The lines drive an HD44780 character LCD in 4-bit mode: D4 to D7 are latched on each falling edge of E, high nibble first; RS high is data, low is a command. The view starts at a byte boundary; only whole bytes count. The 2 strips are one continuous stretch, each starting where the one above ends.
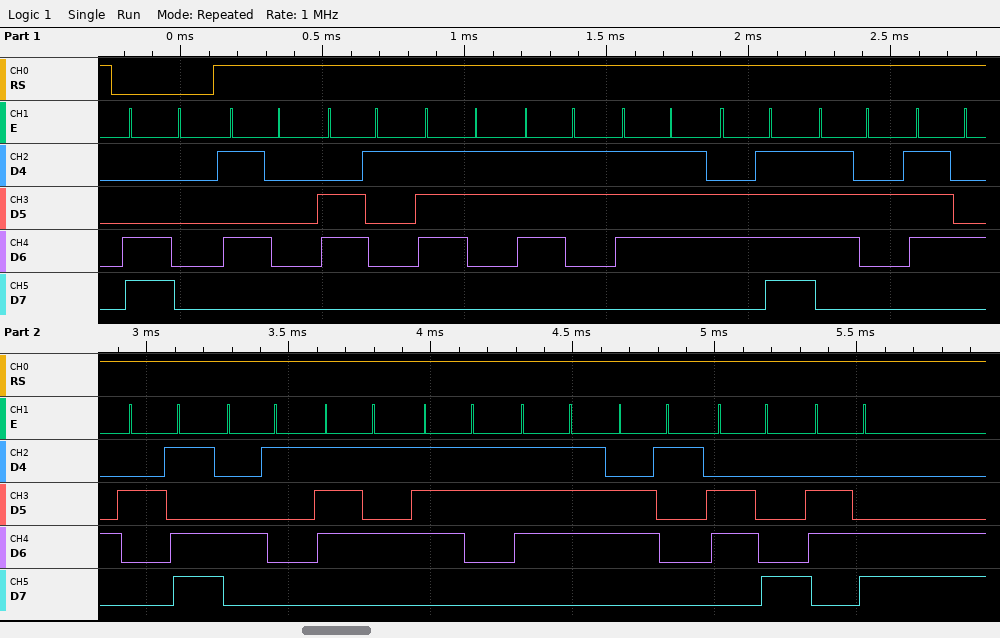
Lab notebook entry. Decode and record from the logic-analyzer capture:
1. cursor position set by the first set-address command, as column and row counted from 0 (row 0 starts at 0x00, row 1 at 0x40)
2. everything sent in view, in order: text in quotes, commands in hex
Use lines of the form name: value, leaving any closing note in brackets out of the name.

cursor position set by the first set-address command, as column and row counted from 0: column 0, row 1
everything sent in view, in order: text in quotes, commands in hex: 0xC0 "Passwort-Auswahl"
